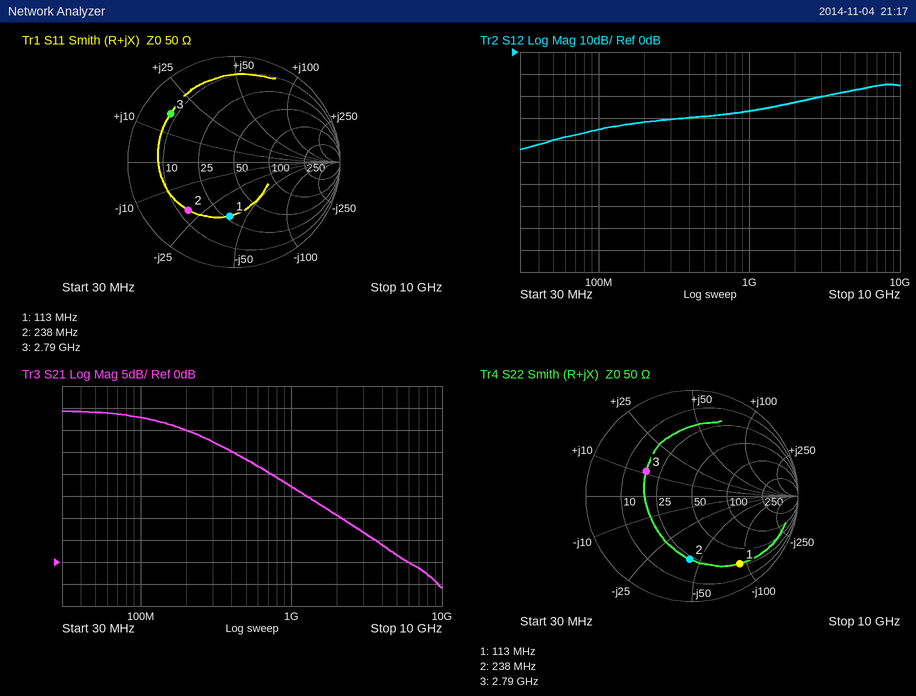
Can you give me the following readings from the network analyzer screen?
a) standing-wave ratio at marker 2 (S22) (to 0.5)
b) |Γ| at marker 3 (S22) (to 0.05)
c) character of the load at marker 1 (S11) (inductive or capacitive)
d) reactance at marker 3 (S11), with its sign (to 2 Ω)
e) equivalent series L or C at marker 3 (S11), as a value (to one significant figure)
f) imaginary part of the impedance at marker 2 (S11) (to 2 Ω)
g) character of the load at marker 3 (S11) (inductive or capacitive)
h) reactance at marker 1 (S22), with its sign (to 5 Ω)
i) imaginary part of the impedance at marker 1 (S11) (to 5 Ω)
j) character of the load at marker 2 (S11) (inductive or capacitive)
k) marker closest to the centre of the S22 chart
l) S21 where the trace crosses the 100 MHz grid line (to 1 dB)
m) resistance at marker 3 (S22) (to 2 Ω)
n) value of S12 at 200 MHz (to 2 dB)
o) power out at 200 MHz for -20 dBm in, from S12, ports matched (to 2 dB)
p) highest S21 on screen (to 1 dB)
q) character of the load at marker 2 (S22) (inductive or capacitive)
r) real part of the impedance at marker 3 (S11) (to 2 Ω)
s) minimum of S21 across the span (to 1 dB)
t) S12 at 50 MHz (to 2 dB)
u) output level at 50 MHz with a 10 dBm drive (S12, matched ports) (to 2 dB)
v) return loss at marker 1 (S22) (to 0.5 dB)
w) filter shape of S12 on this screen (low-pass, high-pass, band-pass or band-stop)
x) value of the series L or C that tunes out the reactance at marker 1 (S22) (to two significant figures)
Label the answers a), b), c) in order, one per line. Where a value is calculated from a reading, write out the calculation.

a) 4.0
b) 0.50
c) capacitive
d) +16 Ω
e) L = 16 Ω/(2π × 2.79 GHz) ≈ 913 pH, so 900 pH to one significant figure
f) -20 Ω
g) inductive
h) -90 Ω
i) -40 Ω
j) capacitive
k) marker 3
l) 33 dB
m) 18 Ω
n) -32 dB
o) -20 dBm + (-32 dB) = -52 dBm
p) 34 dB
q) capacitive
r) 8 Ω
s) -6 dB
t) -40 dB
u) 10 dBm + (-40 dB) = -30 dBm
v) 2.0 dB
w) high-pass
x) L = 90 Ω/(2π × 113 MHz) ≈ 127 nH, so 130 nH to two significant figures
